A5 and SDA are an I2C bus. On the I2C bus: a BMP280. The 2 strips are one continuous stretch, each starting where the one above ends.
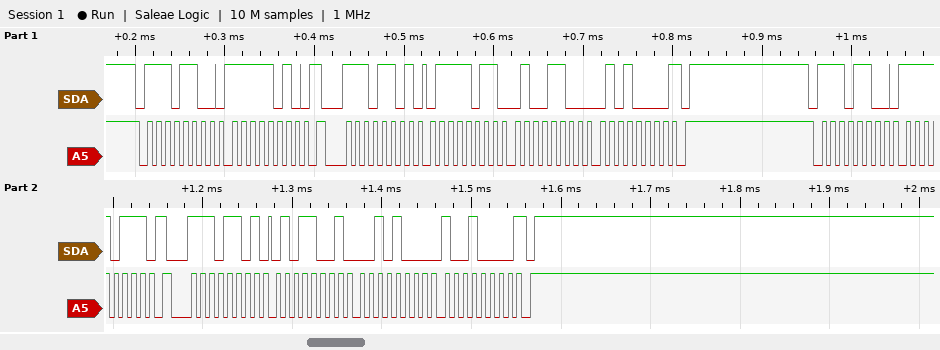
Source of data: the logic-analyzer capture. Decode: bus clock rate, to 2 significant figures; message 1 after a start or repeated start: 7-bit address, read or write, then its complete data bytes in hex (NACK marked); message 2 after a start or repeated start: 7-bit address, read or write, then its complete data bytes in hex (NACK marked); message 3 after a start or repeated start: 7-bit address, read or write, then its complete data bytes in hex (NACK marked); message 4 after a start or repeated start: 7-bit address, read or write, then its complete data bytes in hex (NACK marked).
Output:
100 kHz
0x76 write: FA
0x76 read: 7B 4C 50 NACK
0x76 write: F7
0x76 read: 59 28 90 NACK
